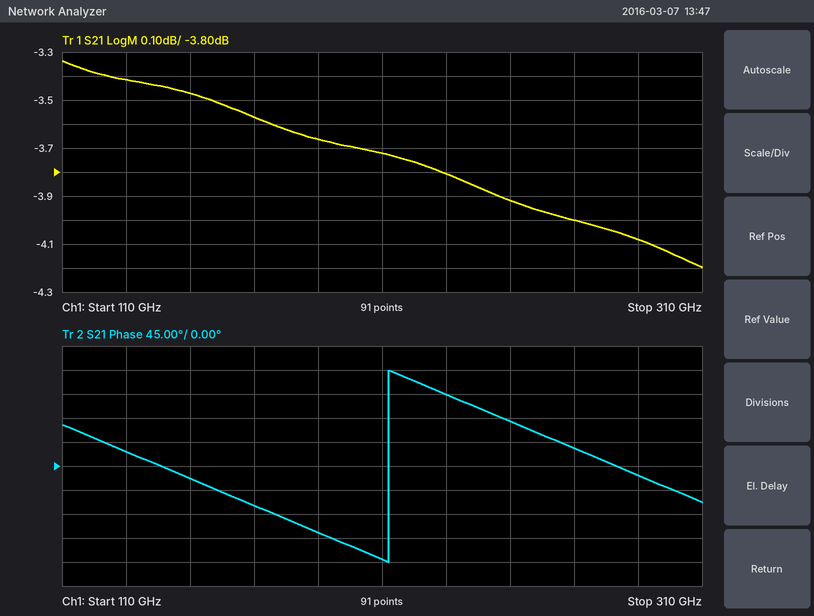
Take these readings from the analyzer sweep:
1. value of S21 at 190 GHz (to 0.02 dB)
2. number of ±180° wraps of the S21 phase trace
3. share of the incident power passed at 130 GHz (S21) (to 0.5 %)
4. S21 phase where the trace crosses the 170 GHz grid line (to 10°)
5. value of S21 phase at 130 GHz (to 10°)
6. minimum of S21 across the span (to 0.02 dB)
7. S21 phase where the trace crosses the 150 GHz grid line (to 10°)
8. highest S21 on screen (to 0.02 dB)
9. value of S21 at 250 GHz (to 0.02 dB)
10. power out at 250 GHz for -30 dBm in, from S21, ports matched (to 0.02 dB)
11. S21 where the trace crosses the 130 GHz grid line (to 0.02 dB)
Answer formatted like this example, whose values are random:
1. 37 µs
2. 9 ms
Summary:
1. -3.66 dB
2. 1
3. 45.5 %
4. -70°
5. 30°
6. -4.20 dB
7. -20°
8. -3.34 dB
9. -3.92 dB
10. -33.92 dBm
11. -3.42 dB
